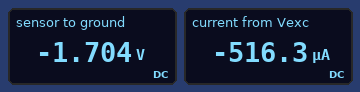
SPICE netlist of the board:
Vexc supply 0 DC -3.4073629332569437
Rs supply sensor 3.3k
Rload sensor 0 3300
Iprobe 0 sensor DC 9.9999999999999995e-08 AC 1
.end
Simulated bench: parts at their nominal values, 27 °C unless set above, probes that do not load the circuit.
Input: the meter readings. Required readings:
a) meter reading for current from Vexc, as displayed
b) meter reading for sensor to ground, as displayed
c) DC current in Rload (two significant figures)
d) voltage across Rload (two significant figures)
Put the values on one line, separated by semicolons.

-516.3 µA; -1.704 V; 520 µA; 1.7 V
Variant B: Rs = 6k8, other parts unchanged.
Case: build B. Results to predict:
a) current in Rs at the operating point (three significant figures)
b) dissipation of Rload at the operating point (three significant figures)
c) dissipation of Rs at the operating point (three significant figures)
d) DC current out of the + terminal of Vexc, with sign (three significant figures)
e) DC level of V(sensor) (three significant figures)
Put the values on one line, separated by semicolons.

337 µA; 375 µW; 774 µW; -337 µA; -1.11 V
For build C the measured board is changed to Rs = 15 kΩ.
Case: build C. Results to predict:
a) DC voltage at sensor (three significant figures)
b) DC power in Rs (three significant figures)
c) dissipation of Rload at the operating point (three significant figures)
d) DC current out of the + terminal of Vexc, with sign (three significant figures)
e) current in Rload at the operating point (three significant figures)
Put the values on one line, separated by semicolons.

-614 mV; 520 µW; 114 µW; -186 µA; 186 µA
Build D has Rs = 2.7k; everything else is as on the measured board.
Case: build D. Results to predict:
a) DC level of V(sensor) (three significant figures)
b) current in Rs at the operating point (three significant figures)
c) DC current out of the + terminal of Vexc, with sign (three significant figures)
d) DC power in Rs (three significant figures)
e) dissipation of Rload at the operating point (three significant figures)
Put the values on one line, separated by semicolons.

-1.87 V; 568 µA; -568 µA; 871 µW; 1.06 mW
